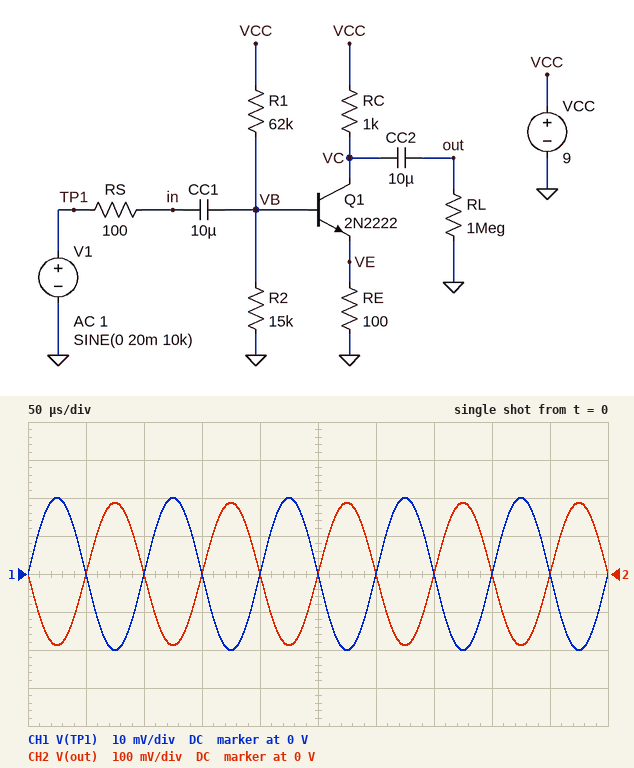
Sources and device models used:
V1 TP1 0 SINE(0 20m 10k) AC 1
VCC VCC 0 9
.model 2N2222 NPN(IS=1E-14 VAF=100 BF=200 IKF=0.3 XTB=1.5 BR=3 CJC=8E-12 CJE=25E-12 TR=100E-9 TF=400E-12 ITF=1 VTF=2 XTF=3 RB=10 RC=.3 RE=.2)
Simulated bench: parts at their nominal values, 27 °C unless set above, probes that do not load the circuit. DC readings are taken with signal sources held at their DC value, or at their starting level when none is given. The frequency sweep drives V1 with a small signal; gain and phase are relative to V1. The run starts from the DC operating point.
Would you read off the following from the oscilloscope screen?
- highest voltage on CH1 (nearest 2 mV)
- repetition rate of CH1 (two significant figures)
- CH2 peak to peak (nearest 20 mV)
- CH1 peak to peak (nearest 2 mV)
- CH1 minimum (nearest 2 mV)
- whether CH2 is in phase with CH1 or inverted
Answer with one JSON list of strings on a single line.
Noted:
["20 mV", "10 kHz", "380 mV", "40 mV", "-20 mV", "inverted"]
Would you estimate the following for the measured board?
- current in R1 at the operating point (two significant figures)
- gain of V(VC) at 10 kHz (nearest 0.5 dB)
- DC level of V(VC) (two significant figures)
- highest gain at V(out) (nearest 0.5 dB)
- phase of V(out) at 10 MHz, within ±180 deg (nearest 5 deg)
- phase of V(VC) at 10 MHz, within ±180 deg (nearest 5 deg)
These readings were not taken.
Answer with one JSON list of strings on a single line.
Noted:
["120 µA", "19.5 dB", "2.5 V", "19.5 dB", "135 deg", "135 deg"]
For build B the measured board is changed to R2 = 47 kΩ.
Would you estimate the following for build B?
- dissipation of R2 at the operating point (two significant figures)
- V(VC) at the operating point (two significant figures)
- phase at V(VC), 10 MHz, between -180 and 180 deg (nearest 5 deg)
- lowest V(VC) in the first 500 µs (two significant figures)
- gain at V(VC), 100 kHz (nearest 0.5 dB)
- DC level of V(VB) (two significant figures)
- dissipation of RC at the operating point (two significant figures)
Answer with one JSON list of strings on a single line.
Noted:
["50 µW", "930 mV", "15 deg", "910 mV", "3.5 dB", "1.5 V", "65 mW"]
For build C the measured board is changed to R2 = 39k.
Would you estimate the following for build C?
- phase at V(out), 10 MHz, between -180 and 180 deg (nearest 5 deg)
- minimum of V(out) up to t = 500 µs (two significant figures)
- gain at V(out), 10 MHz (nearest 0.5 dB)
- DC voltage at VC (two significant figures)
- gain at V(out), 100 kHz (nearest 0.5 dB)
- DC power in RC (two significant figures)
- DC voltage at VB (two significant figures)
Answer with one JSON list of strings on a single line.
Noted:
["20 deg", "-18 mV", "-6.5 dB", "930 mV", "5.0 dB", "65 mW", "1.5 V"]
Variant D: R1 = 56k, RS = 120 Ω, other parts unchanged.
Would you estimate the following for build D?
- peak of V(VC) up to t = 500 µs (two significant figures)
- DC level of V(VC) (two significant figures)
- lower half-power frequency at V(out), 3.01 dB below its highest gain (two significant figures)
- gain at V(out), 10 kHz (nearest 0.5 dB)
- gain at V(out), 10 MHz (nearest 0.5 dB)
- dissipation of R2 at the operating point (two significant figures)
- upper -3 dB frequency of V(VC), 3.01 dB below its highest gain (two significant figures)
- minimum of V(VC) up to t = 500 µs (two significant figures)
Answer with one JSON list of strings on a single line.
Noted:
["1.8 V", "1.6 V", "2.2 Hz", "19.5 dB", "16.0 dB", "140 µW", "8.7 MHz", "1.4 V"]
